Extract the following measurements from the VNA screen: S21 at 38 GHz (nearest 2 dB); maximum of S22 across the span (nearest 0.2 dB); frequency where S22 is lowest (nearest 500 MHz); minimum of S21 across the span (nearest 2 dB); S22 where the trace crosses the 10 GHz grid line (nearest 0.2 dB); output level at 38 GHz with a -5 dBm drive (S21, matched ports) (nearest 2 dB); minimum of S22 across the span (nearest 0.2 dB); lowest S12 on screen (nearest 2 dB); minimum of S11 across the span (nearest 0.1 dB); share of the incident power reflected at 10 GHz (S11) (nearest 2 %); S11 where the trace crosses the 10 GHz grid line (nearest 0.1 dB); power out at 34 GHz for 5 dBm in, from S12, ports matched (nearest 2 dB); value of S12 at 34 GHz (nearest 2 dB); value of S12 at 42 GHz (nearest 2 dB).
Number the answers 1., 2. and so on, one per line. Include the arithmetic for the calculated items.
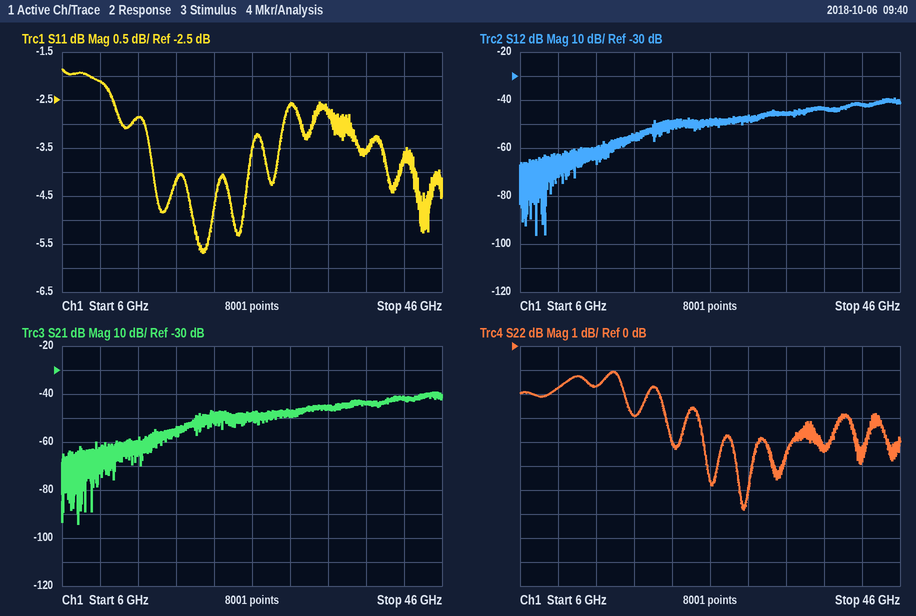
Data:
1. -44 dB
2. -1.0 dB
3. 29.5 GHz
4. -94 dB
5. -1.8 dB
6. -5 dBm + (-44 dB) = -48 dBm
7. -6.8 dB
8. -96 dB
9. -5.7 dB
10. 10^(-2.1/10) ≈ 62 %
11. -2.1 dB
12. 5 dBm + (-46 dB) = -40 dBm
13. -46 dB
14. -42 dB
